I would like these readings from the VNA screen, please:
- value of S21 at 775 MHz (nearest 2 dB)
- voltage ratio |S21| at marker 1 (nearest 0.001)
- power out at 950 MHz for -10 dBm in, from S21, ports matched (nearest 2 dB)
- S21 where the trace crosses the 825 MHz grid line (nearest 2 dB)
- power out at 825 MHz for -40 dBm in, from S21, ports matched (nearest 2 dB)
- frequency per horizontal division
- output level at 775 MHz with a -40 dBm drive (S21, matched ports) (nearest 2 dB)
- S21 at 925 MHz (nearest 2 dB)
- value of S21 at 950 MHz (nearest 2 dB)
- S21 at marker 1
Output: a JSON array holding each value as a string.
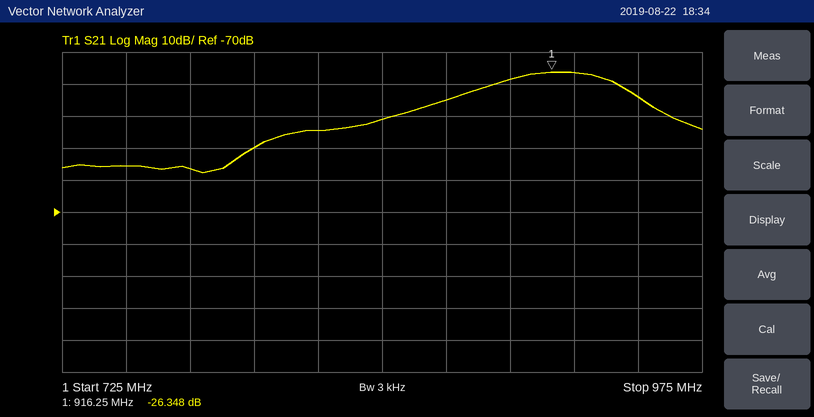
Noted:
["-56 dB", "0.048", "-44 dBm", "-44 dB", "-84 dBm", "25 MHz", "-96 dBm", "-26 dB", "-34 dB", "-26.348 dB"]
